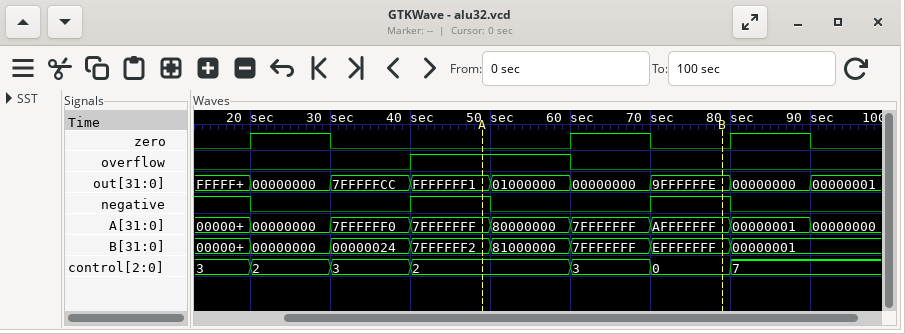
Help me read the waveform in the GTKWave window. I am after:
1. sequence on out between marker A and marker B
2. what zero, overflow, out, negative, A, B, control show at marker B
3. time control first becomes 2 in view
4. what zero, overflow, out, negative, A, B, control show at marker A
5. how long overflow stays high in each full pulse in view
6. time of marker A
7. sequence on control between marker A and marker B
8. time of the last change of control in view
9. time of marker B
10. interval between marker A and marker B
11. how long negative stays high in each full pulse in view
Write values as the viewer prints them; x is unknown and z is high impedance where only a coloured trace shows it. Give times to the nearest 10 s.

FFFFFFF1, 01000000, 00000000, 9FFFFFFE
zero=0, overflow=0, out=9FFFFFFE, negative=1, A=AFFFFFFF, B=EFFFFFFF, control=0
20 s
zero=0, overflow=1, out=FFFFFFF1, negative=1, A=7FFFFFFF, B=7FFFFFF2, control=2
20 s
50 s
2, 3, 0
80 s
80 s
30 s
10 s, 10 s
